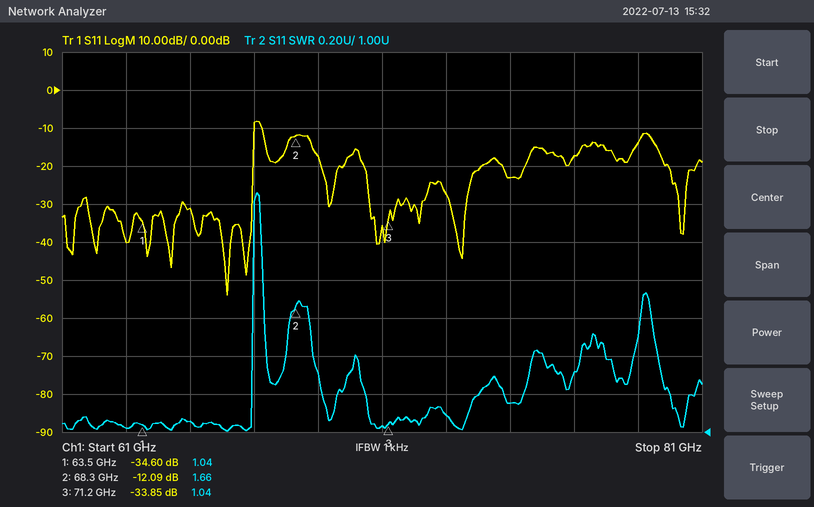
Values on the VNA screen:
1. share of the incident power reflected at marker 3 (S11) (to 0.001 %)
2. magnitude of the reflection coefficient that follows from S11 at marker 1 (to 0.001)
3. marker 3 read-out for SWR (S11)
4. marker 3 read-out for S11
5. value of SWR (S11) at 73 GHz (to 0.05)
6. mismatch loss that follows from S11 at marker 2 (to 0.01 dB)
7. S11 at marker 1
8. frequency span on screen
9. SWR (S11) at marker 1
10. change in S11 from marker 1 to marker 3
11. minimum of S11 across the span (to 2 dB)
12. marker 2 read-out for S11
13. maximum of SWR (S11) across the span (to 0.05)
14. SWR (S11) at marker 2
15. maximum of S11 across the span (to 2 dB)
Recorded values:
0.041 %
0.019
1.04
-33.85 dB
1.10
0.28 dB
-34.60 dB
20 GHz
1.04
0.75 dB
-54 dB
-12.09 dB
2.25
1.66
-8 dB
